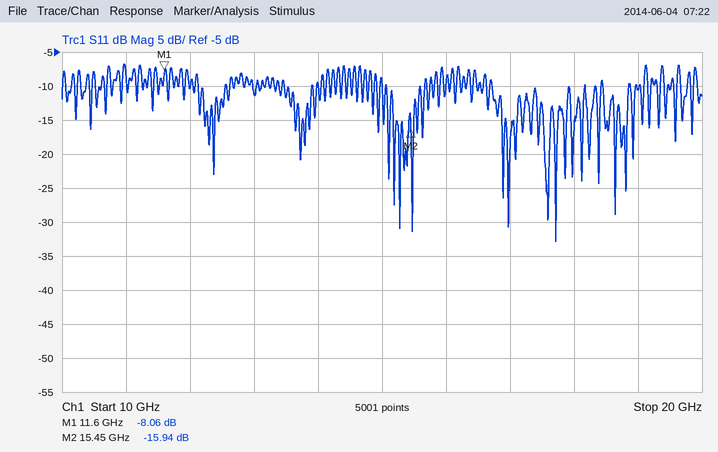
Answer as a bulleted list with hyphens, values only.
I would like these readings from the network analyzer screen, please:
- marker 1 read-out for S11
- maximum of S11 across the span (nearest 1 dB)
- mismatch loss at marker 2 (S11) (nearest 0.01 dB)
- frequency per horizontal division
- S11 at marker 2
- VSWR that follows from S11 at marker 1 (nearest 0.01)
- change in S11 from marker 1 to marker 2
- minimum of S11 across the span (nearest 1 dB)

- -8.06 dB
- -7 dB
- 0.11 dB
- 1 GHz
- -15.94 dB
- 2.31
- -7.88 dB
- -33 dB
